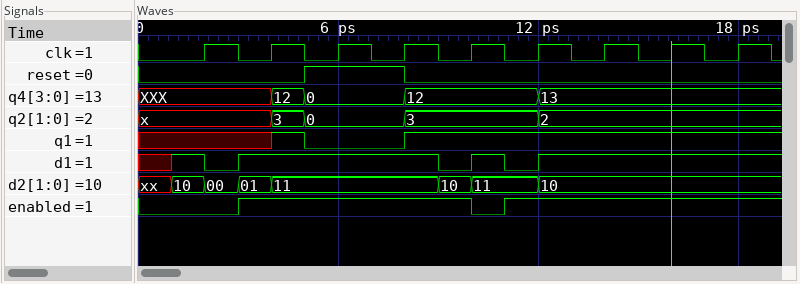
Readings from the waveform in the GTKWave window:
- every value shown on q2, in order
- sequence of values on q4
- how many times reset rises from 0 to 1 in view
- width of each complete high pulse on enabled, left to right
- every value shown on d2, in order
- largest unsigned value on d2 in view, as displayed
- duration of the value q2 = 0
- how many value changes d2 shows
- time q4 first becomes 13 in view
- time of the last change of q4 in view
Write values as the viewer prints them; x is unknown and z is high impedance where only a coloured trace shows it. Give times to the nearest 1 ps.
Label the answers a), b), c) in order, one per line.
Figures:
a) x, 3, 0, 3, 2
b) XXX, 12, 0, 12, 13
c) 1
d) 7 ps
e) xx, 10, 00, 01, 11, 10, 11, 10
f) 11
g) 3 ps
h) 7
i) 12 ps
j) 12 ps
